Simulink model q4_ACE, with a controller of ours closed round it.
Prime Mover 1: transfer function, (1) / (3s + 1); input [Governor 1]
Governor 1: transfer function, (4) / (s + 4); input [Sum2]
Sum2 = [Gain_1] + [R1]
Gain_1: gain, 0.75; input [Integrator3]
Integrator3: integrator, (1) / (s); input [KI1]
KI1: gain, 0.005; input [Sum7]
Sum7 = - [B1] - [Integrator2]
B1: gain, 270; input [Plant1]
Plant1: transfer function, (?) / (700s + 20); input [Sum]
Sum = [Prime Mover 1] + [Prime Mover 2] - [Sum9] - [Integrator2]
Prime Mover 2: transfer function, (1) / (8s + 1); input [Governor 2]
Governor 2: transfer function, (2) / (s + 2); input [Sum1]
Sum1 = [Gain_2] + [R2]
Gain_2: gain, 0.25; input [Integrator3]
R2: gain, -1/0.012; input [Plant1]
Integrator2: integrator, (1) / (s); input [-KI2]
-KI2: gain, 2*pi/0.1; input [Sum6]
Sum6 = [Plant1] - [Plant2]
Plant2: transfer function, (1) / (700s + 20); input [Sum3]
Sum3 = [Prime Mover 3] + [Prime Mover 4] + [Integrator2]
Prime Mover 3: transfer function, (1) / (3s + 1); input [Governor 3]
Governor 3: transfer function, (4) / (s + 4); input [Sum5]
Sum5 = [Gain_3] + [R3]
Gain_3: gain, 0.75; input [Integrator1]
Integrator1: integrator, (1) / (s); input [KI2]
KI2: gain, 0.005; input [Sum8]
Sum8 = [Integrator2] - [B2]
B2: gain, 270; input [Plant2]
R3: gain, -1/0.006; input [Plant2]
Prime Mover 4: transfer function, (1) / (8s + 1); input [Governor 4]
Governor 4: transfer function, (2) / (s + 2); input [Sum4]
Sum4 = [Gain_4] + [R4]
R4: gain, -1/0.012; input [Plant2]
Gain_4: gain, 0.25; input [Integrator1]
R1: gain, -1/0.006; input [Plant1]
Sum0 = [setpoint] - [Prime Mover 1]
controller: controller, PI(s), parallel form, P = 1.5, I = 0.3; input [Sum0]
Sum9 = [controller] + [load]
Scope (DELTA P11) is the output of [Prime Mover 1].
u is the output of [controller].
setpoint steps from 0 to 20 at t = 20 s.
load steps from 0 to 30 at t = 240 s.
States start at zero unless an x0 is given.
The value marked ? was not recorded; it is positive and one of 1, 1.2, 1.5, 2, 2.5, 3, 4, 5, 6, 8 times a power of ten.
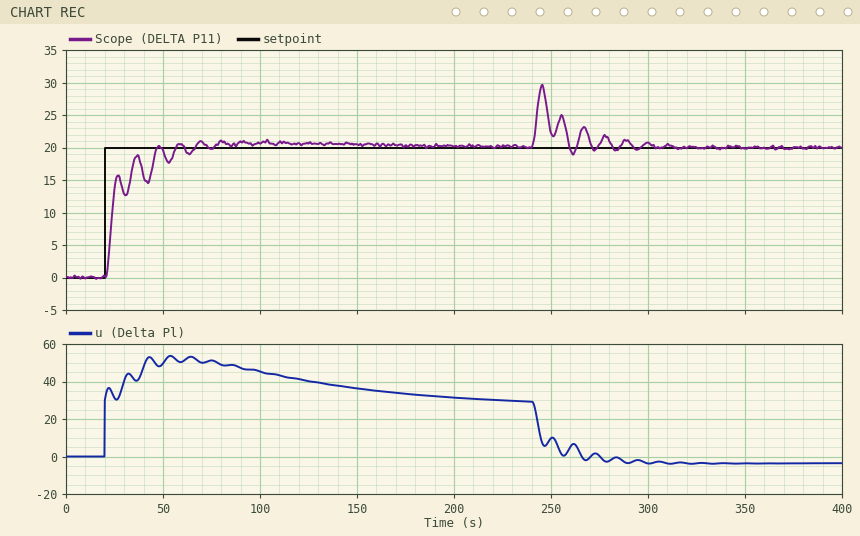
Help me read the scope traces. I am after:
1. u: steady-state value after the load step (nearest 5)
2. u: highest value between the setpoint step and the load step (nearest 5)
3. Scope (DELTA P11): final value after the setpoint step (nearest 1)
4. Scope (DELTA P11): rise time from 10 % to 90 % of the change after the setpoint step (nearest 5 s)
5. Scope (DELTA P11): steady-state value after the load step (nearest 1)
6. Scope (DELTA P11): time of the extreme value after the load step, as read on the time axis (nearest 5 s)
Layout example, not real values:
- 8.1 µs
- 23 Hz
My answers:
- -5
- 55
- 20
- 15 s
- 20
- 245 s
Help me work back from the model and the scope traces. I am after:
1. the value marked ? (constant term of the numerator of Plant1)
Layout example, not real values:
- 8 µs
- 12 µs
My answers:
- 1
